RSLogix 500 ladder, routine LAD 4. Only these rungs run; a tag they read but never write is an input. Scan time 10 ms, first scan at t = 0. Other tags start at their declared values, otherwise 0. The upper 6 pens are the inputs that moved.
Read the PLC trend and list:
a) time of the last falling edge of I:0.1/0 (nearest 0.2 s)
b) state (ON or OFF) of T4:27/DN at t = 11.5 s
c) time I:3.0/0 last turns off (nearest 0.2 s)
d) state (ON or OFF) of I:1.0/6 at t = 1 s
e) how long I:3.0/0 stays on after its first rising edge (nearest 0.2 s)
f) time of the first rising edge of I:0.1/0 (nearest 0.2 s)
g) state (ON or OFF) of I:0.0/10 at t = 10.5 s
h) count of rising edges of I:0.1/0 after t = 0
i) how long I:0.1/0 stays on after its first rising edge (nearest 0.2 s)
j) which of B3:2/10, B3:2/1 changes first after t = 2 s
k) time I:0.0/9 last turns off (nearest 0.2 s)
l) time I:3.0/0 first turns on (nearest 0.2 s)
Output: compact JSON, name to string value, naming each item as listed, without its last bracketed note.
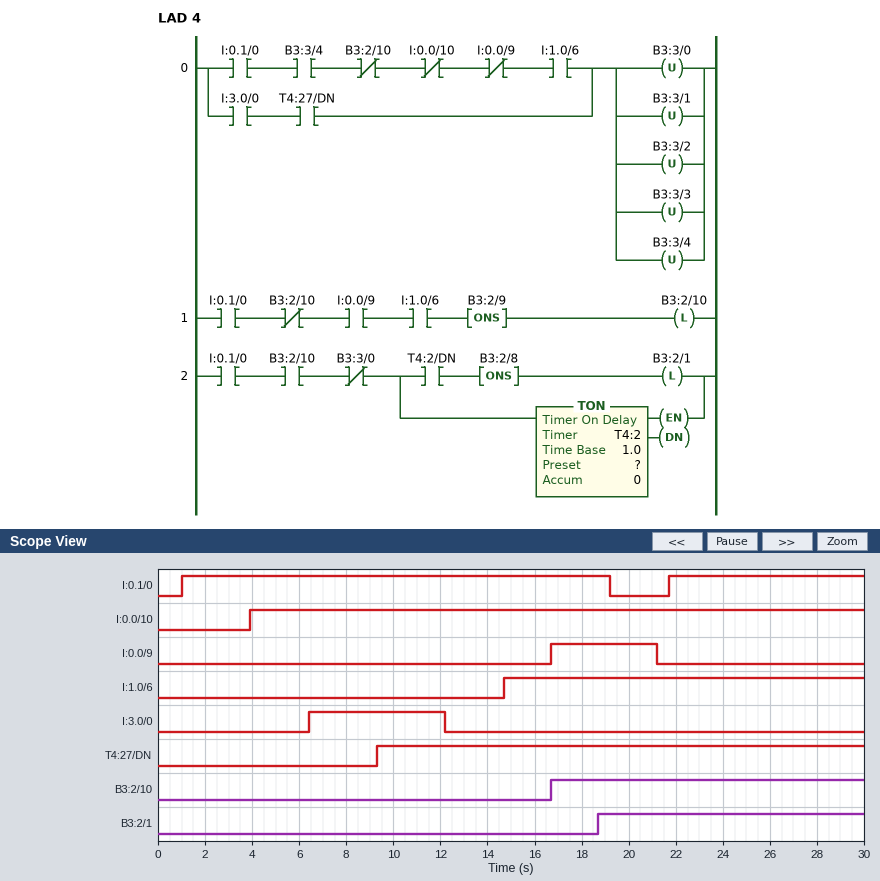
{"time of the last falling edge of I:0.1/0": "19.2 s", "state (ON or OFF) of T4:27/DN at t = 11.5 s": "ON", "time I:3.0/0 last turns off": "12.2 s", "state (ON or OFF) of I:1.0/6 at t = 1 s": "OFF", "how long I:3.0/0 stays on after its first rising edge": "5.8 s", "time of the first rising edge of I:0.1/0": "1.0 s", "state (ON or OFF) of I:0.0/10 at t = 10.5 s": "ON", "count of rising edges of I:0.1/0 after t = 0": "2", "how long I:0.1/0 stays on after its first rising edge": "18.2 s", "which of B3:2/10, B3:2/1 changes first after t = 2 s": "B3:2/10", "time I:0.0/9 last turns off": "21.2 s", "time I:3.0/0 first turns on": "6.4 s"}
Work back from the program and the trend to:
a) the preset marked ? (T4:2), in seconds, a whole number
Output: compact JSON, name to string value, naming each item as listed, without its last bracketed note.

{"the preset marked ? (T4:2), in seconds, a whole number": "2 s"}
